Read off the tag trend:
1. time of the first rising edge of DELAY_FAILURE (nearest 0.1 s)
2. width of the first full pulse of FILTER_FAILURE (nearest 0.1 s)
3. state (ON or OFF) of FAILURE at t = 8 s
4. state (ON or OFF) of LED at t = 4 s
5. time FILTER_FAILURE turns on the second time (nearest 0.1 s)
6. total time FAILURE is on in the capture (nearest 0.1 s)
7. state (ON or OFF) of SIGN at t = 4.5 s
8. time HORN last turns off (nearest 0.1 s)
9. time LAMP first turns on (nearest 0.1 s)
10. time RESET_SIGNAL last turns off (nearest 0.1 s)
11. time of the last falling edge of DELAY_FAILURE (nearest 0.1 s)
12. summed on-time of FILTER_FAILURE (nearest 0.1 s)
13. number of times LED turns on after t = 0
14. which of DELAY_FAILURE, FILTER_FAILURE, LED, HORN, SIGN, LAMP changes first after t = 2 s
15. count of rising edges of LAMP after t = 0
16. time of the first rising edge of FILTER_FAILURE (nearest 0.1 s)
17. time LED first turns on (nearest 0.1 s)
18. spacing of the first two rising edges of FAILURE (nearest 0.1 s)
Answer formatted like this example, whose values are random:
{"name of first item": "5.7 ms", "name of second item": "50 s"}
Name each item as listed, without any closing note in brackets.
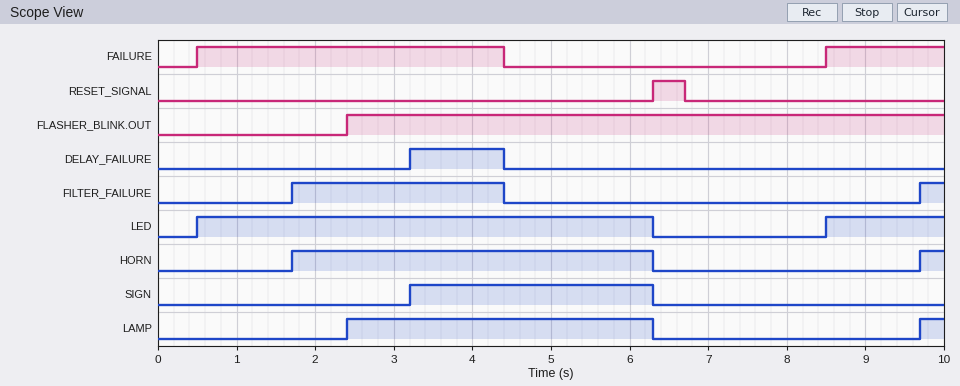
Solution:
{"time of the first rising edge of DELAY_FAILURE": "3.2 s", "width of the first full pulse of FILTER_FAILURE": "2.7 s", "state (ON or OFF) of FAILURE at t = 8 s": "OFF", "state (ON or OFF) of LED at t = 4 s": "ON", "time FILTER_FAILURE turns on the second time": "9.7 s", "total time FAILURE is on in the capture": "5.4 s", "state (ON or OFF) of SIGN at t = 4.5 s": "ON", "time HORN last turns off": "6.3 s", "time LAMP first turns on": "2.4 s", "time RESET_SIGNAL last turns off": "6.7 s", "time of the last falling edge of DELAY_FAILURE": "4.4 s", "summed on-time of FILTER_FAILURE": "3.0 s", "number of times LED turns on after t = 0": "2", "which of DELAY_FAILURE, FILTER_FAILURE, LED, HORN, SIGN, LAMP changes first after t = 2 s": "LAMP", "count of rising edges of LAMP after t = 0": "2", "time of the first rising edge of FILTER_FAILURE": "1.7 s", "time LED first turns on": "0.5 s", "spacing of the first two rising edges of FAILURE": "8.0 s"}
